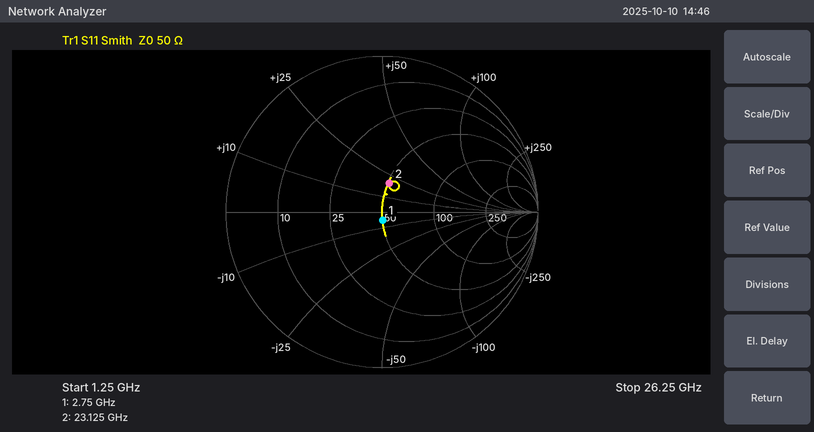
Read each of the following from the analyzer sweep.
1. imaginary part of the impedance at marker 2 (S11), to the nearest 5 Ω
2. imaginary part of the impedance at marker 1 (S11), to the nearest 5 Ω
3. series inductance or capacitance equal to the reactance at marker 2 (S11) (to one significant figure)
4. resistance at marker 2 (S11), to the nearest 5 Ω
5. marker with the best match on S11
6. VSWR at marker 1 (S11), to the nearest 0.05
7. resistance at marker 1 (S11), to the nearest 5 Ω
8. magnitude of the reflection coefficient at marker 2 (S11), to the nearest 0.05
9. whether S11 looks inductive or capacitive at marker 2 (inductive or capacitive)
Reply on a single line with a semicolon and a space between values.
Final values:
+20 Ω; -5 Ω; 100 pH; 50 Ω; marker 1; 1.10; 50 Ω; 0.20; inductive
